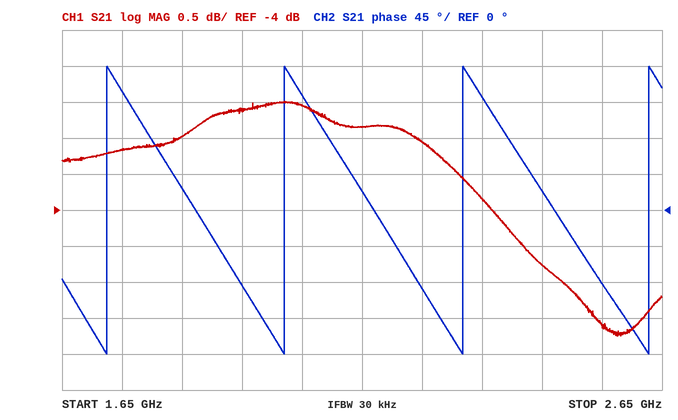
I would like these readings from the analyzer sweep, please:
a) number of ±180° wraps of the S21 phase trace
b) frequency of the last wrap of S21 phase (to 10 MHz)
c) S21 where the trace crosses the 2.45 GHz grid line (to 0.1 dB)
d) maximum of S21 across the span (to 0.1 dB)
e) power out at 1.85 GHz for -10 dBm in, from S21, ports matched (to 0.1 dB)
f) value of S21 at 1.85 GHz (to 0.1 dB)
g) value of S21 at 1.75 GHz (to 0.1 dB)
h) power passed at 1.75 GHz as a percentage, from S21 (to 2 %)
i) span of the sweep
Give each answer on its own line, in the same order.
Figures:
4
2.63 GHz
-4.8 dB
-2.5 dB
-13.0 dBm
-3.0 dB
-3.2 dB
48 %
1 GHz
